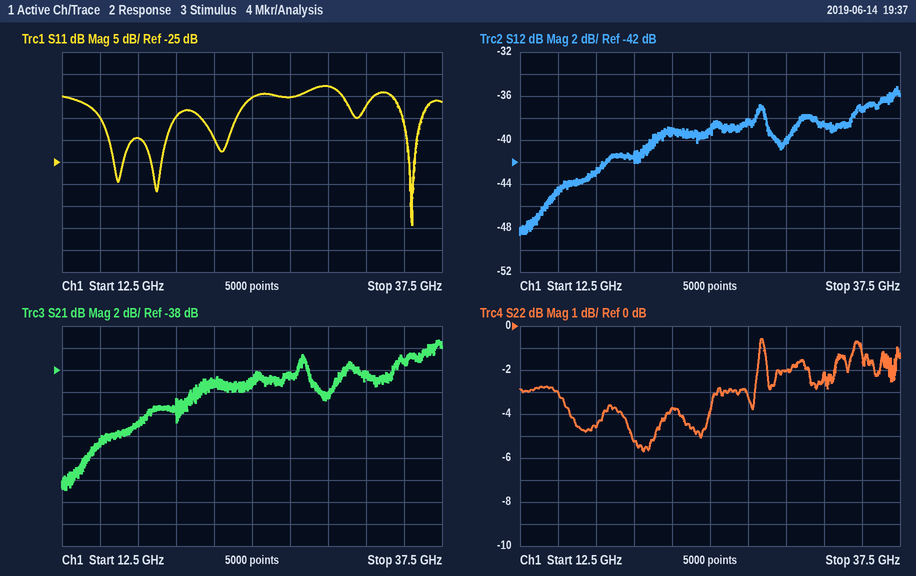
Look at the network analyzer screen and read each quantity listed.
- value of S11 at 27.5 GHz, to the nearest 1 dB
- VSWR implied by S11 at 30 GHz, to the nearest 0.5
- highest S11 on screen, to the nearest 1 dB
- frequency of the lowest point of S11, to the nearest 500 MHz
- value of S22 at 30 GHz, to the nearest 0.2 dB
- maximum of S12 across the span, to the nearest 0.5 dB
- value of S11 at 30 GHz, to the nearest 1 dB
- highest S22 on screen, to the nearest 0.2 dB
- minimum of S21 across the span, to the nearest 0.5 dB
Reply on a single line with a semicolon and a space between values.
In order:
-10 dB; 2.5; -8 dB; 35.5 GHz; -2.0 dB; -35.0 dB; -8 dB; -0.6 dB; -49.0 dB
